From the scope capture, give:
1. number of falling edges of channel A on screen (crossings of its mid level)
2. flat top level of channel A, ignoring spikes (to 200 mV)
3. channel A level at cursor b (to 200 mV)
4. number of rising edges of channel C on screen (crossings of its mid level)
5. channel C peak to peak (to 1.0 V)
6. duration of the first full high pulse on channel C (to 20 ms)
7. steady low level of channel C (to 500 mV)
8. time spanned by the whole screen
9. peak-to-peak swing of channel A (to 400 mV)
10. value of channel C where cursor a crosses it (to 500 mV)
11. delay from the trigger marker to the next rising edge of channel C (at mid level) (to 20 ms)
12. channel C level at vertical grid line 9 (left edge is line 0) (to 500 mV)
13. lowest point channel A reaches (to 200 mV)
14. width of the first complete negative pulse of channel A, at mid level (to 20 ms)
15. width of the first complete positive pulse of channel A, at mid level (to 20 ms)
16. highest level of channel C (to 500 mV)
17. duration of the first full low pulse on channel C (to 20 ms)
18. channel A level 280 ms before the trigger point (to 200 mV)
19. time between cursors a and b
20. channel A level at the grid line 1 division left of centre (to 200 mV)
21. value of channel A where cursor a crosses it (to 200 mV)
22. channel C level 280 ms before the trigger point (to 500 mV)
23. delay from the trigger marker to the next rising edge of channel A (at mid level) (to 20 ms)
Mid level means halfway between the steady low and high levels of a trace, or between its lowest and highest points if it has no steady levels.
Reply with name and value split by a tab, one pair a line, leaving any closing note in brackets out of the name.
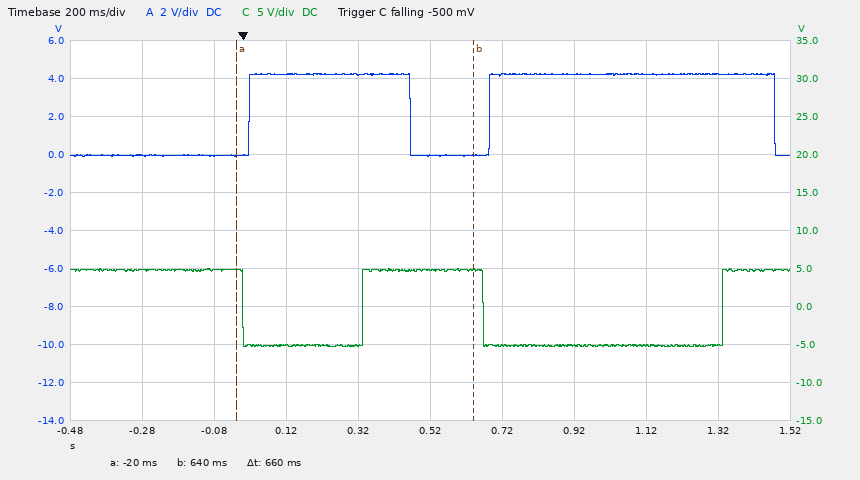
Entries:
number of falling edges of channel A on screen	2
flat top level of channel A, ignoring spikes	4.2 V
channel A level at cursor b	0.0 V
number of rising edges of channel C on screen	2
channel C peak to peak	10.0 V
duration of the first full high pulse on channel C	340 ms
steady low level of channel C	-5.0 V
time spanned by the whole screen	2 s
peak-to-peak swing of channel A	4.4 V
value of channel C where cursor a crosses it	5.0 V
delay from the trigger marker to the next rising edge of channel C (at mid level)	340 ms
channel C level at vertical grid line 9 (left edge is line 0)	-5.0 V
lowest point channel A reaches	-200 mV
width of the first complete negative pulse of channel A, at mid level	220 ms
width of the first complete positive pulse of channel A, at mid level	440 ms
highest level of channel C	5.0 V
duration of the first full low pulse on channel C	340 ms
channel A level 280 ms before the trigger point	0.0 V
time between cursors a and b	660 ms
channel A level at the grid line 1 division left of centre	4.2 V
value of channel A where cursor a crosses it	0.0 V
channel C level 280 ms before the trigger point	5.0 V
delay from the trigger marker to the next rising edge of channel A (at mid level)	20 ms
